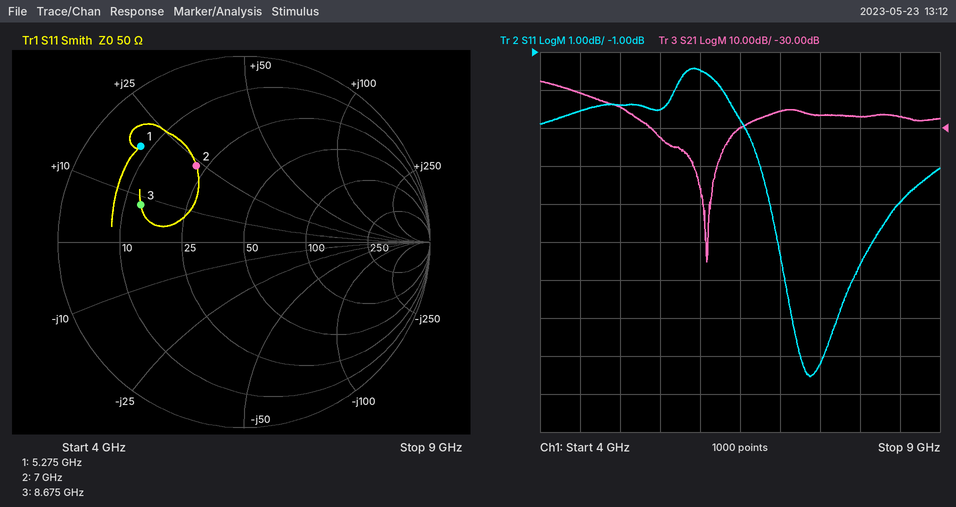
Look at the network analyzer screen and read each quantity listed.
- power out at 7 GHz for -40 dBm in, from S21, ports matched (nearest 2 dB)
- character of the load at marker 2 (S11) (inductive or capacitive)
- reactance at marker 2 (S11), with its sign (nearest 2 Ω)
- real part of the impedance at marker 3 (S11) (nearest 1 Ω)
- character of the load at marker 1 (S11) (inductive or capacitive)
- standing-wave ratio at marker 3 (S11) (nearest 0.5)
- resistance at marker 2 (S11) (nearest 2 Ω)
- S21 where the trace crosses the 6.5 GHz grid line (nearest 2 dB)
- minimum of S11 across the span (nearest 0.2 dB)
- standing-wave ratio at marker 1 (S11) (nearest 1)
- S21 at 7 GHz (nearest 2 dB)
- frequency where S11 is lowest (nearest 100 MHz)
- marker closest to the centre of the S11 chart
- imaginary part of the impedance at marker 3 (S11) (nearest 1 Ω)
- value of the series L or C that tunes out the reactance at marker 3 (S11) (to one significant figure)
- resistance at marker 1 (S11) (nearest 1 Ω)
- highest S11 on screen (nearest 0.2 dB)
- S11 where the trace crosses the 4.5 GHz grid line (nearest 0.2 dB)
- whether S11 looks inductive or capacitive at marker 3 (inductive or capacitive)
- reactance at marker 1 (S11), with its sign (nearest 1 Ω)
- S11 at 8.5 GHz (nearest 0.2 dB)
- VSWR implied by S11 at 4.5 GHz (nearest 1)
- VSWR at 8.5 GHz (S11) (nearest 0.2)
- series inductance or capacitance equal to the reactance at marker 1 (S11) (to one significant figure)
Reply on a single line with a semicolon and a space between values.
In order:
-66 dBm; inductive; +24 Ω; 13 Ω; inductive; 4.0; 22 Ω; -30 dB; -9.6 dB; 7; -26 dB; 7.4 GHz; marker 2; +8 Ω; 2 pF; 8 Ω; -1.4 dB; -2.6 dB; inductive; +19 Ω; -5.0 dB; 7; 3.6; 600 pH
